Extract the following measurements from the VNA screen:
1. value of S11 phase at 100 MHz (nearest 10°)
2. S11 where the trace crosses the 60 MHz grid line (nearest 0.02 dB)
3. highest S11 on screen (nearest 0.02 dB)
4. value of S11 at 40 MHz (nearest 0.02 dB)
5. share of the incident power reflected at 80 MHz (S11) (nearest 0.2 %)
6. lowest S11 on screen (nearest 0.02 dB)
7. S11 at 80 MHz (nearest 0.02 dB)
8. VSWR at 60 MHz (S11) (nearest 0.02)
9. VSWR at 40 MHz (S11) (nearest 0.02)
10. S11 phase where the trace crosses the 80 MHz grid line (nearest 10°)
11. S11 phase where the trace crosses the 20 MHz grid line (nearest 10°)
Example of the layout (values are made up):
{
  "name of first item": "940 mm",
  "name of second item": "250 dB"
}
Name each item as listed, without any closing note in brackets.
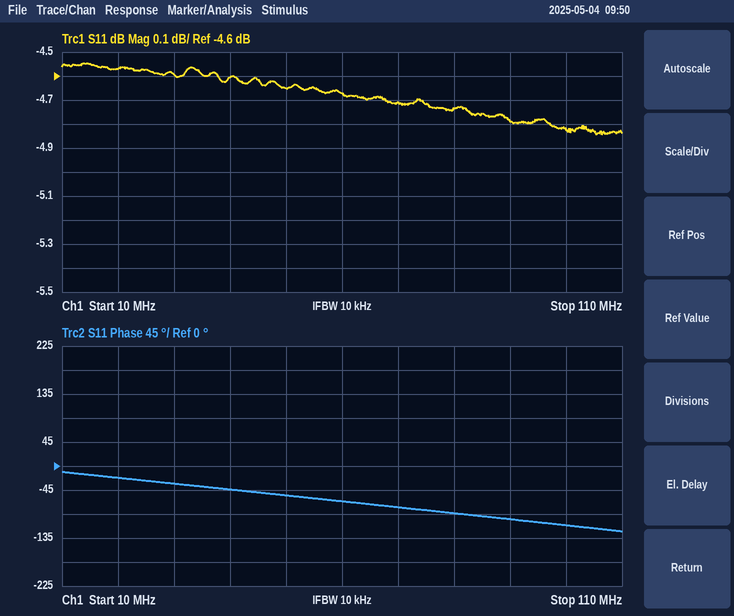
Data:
{
  "value of S11 phase at 100 MHz": "-110°",
  "S11 where the trace crosses the 60 MHz grid line": "-4.68 dB",
  "highest S11 on screen": "-4.54 dB",
  "value of S11 at 40 MHz": "-4.60 dB",
  "share of the incident power reflected at 80 MHz (S11)": "33.6 %",
  "lowest S11 on screen": "-4.84 dB",
  "S11 at 80 MHz": "-4.74 dB",
  "VSWR at 60 MHz (S11)": "3.80",
  "VSWR at 40 MHz (S11)": "3.86",
  "S11 phase where the trace crosses the 80 MHz grid line": "-90°",
  "S11 phase where the trace crosses the 20 MHz grid line": "-20°"
}
